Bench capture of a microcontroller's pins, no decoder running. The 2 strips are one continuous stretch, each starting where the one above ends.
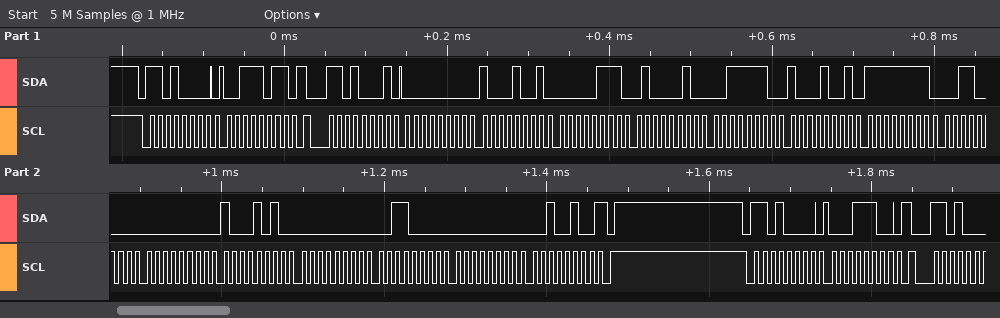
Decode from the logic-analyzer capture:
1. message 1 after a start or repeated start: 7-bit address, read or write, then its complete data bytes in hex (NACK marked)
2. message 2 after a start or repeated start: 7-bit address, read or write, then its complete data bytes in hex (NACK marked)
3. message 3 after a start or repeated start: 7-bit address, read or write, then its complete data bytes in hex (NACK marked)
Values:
0x68 write: 3B
0x68 read: 00 89 07 42 3E 89 FF 30 00 8A 00 30 00 24 NACK
0x68 write: 1C
